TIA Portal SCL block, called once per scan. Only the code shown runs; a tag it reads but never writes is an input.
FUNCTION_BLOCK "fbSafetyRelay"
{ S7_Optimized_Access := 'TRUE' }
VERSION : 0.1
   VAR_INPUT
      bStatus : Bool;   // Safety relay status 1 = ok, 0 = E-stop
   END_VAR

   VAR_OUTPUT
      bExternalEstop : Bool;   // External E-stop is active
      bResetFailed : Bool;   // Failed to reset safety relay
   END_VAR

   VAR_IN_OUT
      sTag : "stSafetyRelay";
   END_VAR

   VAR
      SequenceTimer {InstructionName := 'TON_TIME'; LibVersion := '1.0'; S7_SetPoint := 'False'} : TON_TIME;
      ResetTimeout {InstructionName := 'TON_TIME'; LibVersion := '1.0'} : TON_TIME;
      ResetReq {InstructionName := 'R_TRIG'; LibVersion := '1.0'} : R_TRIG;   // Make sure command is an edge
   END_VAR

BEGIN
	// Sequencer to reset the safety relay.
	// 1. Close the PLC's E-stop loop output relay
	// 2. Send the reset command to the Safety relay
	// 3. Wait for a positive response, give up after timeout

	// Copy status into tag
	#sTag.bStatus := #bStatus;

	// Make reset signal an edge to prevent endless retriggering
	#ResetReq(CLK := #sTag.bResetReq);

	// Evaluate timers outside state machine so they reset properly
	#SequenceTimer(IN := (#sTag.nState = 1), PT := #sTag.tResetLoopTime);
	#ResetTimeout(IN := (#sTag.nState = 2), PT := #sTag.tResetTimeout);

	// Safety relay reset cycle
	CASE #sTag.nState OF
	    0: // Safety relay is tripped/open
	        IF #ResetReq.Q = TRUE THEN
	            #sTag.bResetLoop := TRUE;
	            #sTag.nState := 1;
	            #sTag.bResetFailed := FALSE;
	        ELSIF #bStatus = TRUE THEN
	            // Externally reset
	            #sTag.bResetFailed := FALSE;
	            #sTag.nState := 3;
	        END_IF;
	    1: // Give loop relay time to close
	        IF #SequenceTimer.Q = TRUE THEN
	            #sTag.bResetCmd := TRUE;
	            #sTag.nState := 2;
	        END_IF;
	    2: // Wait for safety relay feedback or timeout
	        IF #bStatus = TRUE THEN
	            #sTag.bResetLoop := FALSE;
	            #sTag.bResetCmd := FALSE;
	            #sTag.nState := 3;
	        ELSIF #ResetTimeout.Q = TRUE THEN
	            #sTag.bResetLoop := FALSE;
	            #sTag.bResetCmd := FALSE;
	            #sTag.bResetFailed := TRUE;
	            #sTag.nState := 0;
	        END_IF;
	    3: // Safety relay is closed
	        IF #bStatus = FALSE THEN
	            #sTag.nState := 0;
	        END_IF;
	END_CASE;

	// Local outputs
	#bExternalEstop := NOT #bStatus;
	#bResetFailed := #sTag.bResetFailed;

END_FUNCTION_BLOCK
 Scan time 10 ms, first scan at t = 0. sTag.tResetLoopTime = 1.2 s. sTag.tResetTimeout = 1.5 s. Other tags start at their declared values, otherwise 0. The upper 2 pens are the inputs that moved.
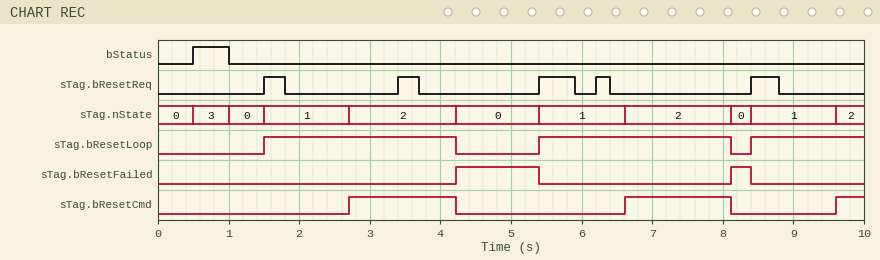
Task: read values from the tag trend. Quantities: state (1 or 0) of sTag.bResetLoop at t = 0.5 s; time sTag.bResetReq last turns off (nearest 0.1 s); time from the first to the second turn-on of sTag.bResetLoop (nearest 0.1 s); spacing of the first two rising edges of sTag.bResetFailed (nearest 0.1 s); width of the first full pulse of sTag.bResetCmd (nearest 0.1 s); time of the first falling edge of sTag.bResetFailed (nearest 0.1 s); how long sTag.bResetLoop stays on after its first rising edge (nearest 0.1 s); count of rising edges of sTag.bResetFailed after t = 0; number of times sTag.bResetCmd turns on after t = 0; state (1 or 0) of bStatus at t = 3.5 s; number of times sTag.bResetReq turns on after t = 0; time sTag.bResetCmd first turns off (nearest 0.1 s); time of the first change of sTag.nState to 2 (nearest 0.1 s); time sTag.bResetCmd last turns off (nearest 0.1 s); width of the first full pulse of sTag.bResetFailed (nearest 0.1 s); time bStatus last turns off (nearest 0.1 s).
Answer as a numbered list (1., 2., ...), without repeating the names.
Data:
1. 0
2. 8.8 s
3. 3.9 s
4. 3.9 s
5. 1.5 s
6. 5.4 s
7. 2.7 s
8. 2
9. 3
10. 0
11. 5
12. 4.2 s
13. 2.7 s
14. 8.1 s
15. 1.2 s
16. 1.0 s
